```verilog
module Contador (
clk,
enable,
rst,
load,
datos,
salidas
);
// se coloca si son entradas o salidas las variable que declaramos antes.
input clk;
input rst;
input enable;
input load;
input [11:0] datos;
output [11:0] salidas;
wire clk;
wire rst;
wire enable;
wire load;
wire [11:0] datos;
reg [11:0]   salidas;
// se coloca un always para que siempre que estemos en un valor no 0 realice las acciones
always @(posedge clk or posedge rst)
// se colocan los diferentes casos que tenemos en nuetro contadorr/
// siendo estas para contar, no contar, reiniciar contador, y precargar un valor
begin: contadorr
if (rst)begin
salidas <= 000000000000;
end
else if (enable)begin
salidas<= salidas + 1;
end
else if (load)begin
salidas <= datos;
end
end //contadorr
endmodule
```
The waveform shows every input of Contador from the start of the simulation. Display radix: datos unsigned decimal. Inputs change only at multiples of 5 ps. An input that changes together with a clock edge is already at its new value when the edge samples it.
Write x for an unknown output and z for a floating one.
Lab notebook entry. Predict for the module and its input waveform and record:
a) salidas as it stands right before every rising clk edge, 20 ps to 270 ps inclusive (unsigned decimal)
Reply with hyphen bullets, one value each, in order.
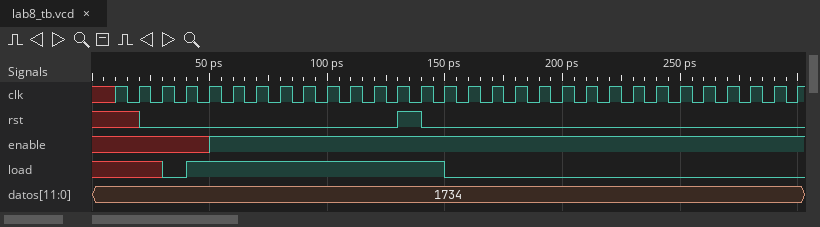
- x, x, x, 1734, 1735, 1736, 1737, 1738, 1739, 1740, 1741, 1742, 0, 1, 2, 3, 4, 5, 6, 7, 8, 9, 10, 11, 12, 13
